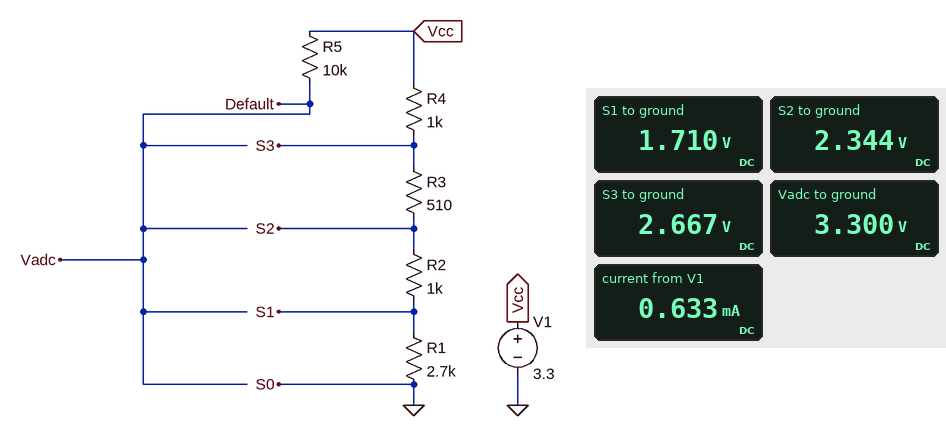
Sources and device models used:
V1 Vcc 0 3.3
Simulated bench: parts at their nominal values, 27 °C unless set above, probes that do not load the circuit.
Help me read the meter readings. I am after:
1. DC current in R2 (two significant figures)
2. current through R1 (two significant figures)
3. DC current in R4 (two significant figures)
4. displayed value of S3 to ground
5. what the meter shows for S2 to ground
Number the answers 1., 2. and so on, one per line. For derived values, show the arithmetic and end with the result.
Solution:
1. (2.344 V - 1.71 V) / 1 kΩ = 630 µA
2. (1.71 V) / 2.7 kΩ = 630 µA
3. (3.3 V - 2.667 V) / 1 kΩ = 630 µA
4. 2.667 V
5. 2.344 V
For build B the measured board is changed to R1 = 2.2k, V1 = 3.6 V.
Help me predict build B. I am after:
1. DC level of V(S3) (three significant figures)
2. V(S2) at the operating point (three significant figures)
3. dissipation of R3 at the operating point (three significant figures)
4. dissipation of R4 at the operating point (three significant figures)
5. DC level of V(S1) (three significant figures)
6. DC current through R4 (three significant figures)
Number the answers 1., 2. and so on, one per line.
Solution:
1. 2.84 V
2. 2.45 V
3. 298 µW
4. 584 µW
5. 1.68 V
6. 764 µA
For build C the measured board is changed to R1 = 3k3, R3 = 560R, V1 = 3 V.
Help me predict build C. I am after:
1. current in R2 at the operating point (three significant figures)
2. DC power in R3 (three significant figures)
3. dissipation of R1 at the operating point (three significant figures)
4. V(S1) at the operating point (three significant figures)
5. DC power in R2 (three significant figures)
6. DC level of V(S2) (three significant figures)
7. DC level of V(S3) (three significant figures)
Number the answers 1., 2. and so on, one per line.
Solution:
1. 512 µA
2. 147 µW
3. 865 µW
4. 1.69 V
5. 262 µW
6. 2.20 V
7. 2.49 V
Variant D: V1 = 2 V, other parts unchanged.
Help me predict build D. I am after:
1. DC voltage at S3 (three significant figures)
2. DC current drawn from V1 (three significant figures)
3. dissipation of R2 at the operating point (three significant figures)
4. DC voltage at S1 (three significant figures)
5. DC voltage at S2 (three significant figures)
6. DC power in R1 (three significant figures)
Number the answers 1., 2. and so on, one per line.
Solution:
1. 1.62 V
2. 384 µA
3. 147 µW
4. 1.04 V
5. 1.42 V
6. 398 µW
